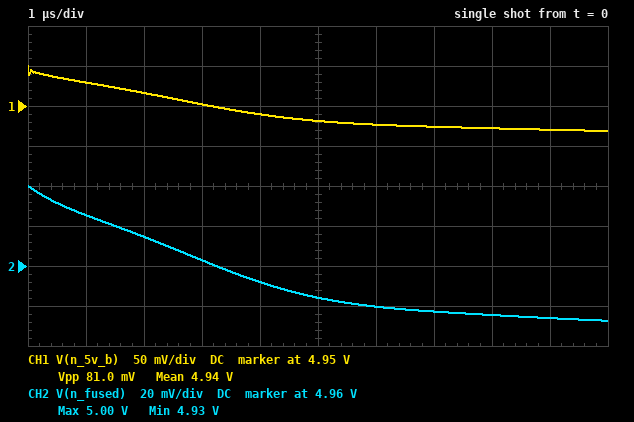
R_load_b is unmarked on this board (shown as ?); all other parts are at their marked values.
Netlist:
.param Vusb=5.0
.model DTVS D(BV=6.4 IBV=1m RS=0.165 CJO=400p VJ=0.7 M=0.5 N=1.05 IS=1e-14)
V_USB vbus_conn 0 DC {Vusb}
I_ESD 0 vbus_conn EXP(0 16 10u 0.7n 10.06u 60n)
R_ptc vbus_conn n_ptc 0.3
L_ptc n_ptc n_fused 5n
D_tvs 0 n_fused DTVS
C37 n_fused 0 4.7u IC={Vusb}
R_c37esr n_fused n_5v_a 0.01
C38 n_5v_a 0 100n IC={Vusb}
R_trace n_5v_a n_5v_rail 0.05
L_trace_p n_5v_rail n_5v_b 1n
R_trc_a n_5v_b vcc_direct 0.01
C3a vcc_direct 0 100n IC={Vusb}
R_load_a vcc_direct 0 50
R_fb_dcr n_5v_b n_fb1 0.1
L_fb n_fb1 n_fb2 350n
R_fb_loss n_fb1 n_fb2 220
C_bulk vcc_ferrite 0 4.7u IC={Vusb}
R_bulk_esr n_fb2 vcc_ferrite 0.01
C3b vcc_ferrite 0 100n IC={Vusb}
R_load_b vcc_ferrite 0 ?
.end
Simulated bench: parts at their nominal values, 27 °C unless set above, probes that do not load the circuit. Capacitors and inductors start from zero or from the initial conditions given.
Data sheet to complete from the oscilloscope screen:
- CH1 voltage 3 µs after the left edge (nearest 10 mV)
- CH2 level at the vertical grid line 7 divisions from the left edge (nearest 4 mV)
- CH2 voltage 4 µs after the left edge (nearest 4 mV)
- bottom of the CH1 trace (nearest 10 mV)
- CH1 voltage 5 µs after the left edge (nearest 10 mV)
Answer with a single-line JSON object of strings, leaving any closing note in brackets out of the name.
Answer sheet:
{"CH1 voltage 3 µs after the left edge": "4.95 V", "CH2 level at the vertical grid line 7 divisions from the left edge": "4.936 V", "CH2 voltage 4 µs after the left edge": "4.952 V", "bottom of the CH1 trace": "4.92 V", "CH1 voltage 5 µs after the left edge": "4.93 V"}
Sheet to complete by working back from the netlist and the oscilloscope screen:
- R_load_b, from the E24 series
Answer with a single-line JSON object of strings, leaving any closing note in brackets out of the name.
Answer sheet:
{"R_load_b, from the E24 series": "36 Ω"}
